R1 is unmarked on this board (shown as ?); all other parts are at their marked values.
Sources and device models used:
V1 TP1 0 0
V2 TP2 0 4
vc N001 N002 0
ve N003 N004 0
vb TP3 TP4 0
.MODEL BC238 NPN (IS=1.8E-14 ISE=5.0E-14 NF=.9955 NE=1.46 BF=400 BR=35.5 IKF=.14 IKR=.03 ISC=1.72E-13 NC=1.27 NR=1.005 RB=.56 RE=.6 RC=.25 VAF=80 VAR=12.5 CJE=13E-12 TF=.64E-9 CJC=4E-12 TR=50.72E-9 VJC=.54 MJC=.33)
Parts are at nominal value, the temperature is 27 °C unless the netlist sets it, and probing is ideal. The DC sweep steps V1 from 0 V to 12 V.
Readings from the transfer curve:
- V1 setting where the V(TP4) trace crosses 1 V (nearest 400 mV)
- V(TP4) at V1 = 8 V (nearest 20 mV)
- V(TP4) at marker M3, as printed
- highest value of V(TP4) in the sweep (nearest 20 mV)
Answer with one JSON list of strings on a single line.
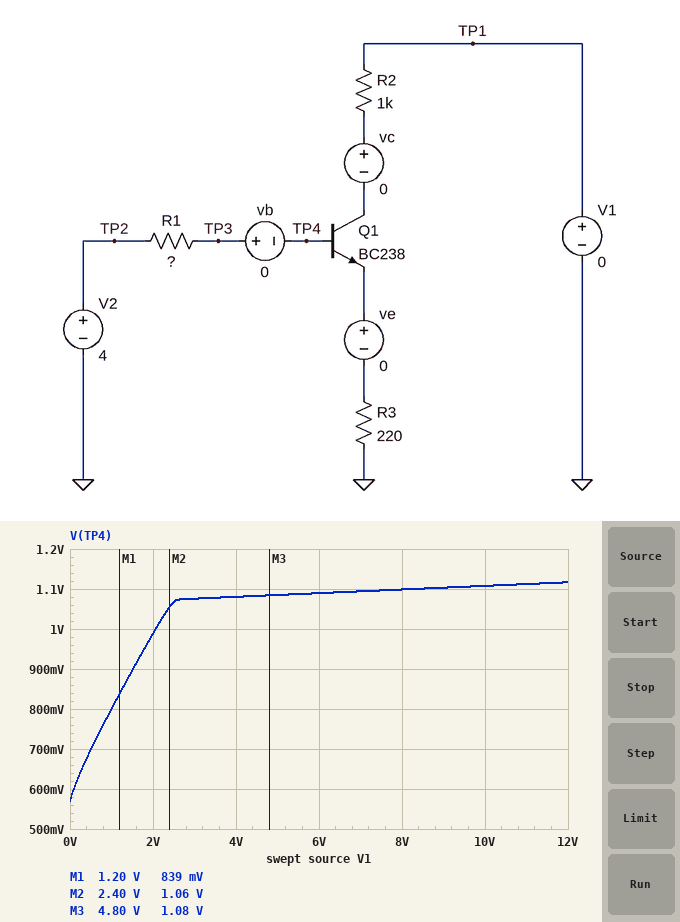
["2.0 V", "1.10 V", "1.08 V", "1.12 V"]
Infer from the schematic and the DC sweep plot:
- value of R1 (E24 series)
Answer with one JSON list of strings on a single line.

["430 kΩ"]
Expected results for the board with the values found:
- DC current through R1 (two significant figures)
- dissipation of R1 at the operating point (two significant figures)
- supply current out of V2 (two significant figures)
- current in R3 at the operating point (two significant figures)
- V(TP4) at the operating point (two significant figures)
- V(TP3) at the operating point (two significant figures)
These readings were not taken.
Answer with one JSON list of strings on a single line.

["8.0 µA", "27 µW", "8.0 µA", "8.2 µA", "570 mV", "570 mV"]
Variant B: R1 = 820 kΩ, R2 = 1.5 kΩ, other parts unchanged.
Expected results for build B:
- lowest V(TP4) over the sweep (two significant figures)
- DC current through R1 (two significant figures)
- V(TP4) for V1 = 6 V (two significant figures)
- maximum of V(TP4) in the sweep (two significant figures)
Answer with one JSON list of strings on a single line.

["550 mV", "4.2 µA", "870 mV", "890 mV"]
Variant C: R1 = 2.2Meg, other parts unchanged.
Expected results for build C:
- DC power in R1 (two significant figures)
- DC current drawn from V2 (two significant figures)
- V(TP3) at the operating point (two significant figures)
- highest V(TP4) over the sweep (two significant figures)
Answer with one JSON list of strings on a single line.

["5.5 µW", "1.6 µA", "520 mV", "700 mV"]
